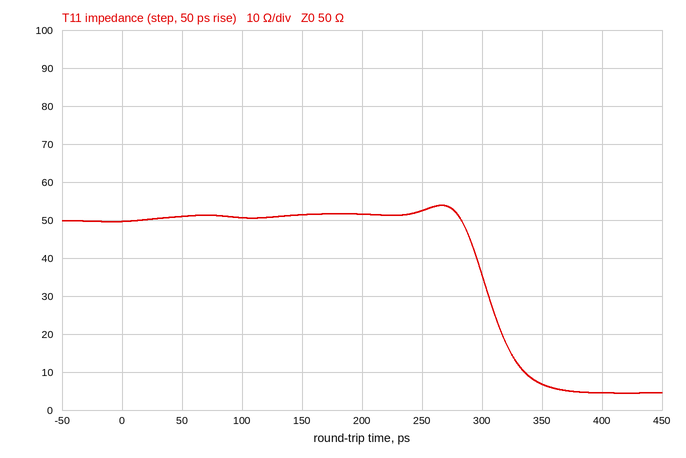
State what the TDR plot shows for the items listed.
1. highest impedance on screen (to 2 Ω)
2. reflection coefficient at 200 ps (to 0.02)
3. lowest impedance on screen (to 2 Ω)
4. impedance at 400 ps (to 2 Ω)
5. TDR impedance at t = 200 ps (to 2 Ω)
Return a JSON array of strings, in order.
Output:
["54 Ω", "+0.02", "4 Ω", "4 Ω", "52 Ω"]
